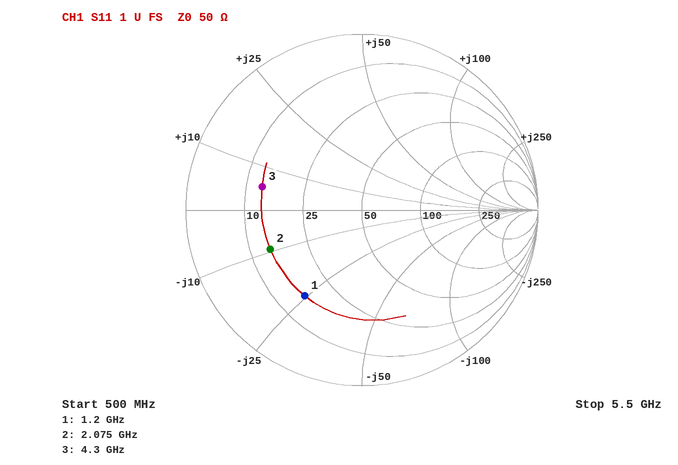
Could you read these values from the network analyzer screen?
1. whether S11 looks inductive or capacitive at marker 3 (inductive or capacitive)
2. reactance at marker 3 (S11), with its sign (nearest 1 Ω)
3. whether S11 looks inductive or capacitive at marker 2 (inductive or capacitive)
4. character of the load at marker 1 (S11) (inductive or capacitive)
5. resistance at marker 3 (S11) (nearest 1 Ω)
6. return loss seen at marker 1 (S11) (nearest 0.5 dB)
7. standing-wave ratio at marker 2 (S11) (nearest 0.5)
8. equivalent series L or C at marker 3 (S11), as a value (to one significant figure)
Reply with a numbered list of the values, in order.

1. inductive
2. +5 Ω
3. capacitive
4. capacitive
5. 13 Ω
6. 4.5 dB
7. 3.5
8. 200 pH
